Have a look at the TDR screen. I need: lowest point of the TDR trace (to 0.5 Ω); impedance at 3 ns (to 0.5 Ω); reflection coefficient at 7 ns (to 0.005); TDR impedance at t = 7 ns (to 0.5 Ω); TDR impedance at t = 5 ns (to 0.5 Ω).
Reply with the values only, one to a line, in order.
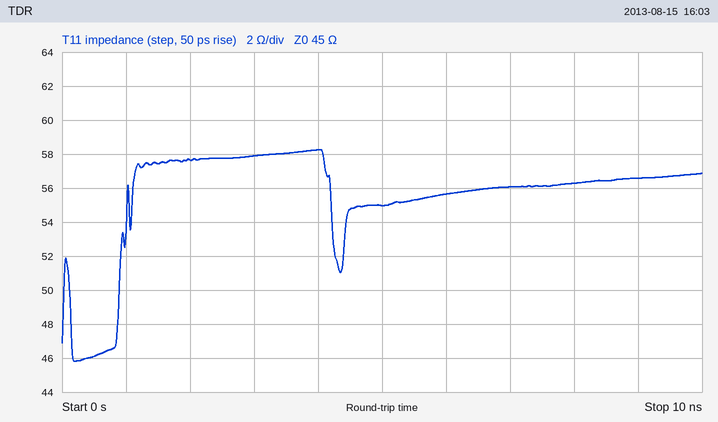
46.0 Ω
58.0 Ω
+0.110
56.0 Ω
55.0 Ω
